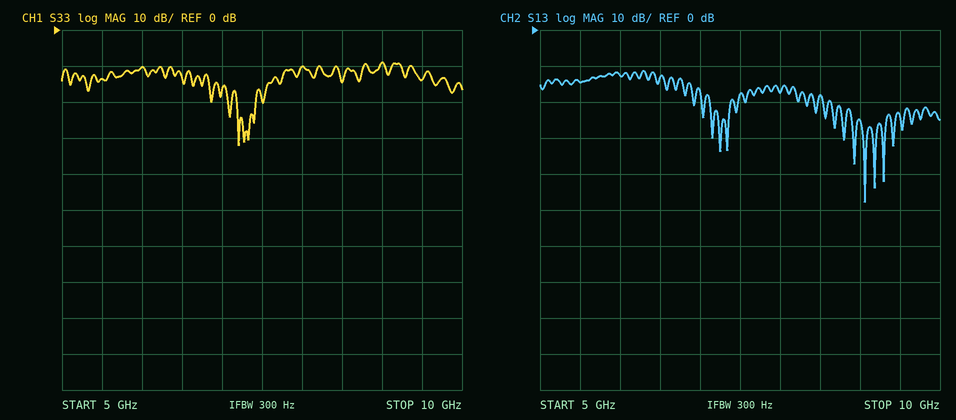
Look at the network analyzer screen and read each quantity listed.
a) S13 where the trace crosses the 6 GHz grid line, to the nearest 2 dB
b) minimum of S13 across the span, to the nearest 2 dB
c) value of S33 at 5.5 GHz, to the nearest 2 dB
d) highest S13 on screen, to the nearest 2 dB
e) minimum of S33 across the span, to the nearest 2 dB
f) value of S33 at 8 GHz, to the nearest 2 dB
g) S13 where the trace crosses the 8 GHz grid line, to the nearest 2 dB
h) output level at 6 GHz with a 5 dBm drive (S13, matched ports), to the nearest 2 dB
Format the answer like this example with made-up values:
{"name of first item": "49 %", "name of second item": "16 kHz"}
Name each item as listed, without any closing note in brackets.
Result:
{"S13 where the trace crosses the 6 GHz grid line, to the nearest 2 dB": "-12 dB", "minimum of S13 across the span, to the nearest 2 dB": "-48 dB", "value of S33 at 5.5 GHz, to the nearest 2 dB": "-14 dB", "highest S13 on screen, to the nearest 2 dB": "-12 dB", "minimum of S33 across the span, to the nearest 2 dB": "-32 dB", "value of S33 at 8 GHz, to the nearest 2 dB": "-10 dB", "S13 where the trace crosses the 8 GHz grid line, to the nearest 2 dB": "-18 dB", "output level at 6 GHz with a 5 dBm drive (S13, matched ports), to the nearest 2 dB": "-8 dBm"}
